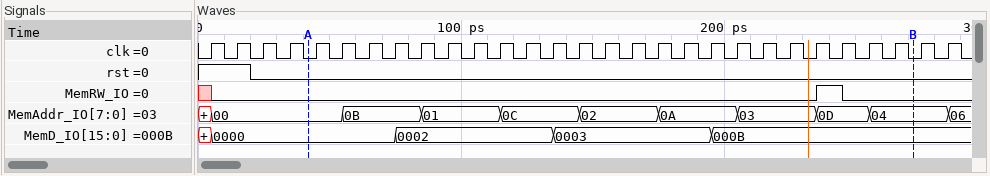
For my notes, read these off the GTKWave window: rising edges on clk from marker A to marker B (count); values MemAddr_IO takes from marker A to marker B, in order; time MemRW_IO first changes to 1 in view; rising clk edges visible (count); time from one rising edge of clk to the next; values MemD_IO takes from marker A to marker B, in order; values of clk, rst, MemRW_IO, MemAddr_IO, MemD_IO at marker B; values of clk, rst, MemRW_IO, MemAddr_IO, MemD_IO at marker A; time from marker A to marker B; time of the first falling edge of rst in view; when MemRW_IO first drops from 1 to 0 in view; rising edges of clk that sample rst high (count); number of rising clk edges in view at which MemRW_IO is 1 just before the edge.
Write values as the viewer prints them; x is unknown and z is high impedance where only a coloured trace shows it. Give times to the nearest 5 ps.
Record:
23
00, 0B, 01, 0C, 02, 0A, 03, 0D, 04
235 ps
29
10 ps
0000, 0002, 0003, 000B
clk=0, rst=0, MemRW_IO=0, MemAddr_IO=04, MemD_IO=000B
clk=0, rst=0, MemRW_IO=0, MemAddr_IO=00, MemD_IO=0000
230 ps
20 ps
245 ps
2
1
